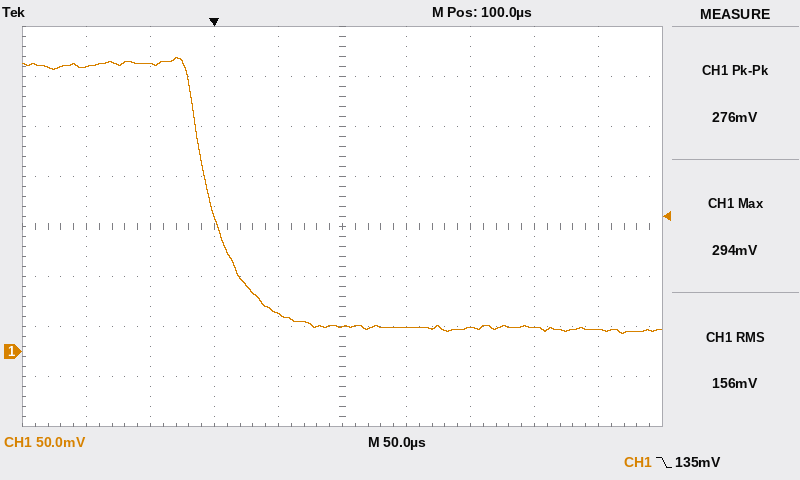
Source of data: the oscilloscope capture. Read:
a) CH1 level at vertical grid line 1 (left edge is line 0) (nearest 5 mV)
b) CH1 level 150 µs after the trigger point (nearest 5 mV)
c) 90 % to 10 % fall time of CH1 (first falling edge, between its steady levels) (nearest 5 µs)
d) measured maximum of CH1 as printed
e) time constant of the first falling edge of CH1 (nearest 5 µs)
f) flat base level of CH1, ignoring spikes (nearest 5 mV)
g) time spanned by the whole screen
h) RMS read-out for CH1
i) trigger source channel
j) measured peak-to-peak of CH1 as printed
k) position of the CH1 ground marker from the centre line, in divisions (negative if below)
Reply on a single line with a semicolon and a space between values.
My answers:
285 mV; 25 mV; 55 µs; 294 mV; 25 µs; 25 mV; 500 µs; 156 mV; CH1; 276 mV; -2.5 div
